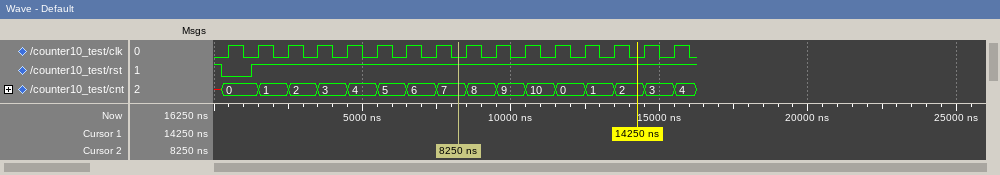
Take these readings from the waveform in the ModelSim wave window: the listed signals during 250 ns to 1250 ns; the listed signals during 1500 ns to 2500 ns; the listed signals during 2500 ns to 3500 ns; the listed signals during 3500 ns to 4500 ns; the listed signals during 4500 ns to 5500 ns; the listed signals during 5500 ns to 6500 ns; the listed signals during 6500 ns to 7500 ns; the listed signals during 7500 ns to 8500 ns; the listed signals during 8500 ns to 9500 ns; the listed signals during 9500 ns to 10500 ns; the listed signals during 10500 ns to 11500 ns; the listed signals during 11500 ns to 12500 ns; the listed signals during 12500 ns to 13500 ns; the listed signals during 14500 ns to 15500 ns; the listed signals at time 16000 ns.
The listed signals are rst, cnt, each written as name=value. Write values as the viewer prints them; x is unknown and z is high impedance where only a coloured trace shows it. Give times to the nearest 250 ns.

rst=0, cnt=0
rst=1, cnt=1
rst=1, cnt=2
rst=1, cnt=3
rst=1, cnt=4
rst=1, cnt=5
rst=1, cnt=6
rst=1, cnt=7
rst=1, cnt=8
rst=1, cnt=9
rst=1, cnt=10
rst=1, cnt=0
rst=1, cnt=1
rst=1, cnt=3
rst=1, cnt=4
